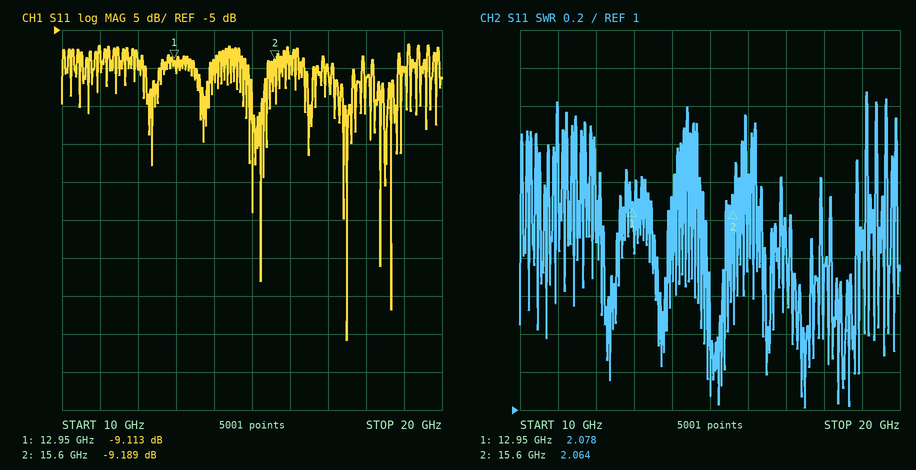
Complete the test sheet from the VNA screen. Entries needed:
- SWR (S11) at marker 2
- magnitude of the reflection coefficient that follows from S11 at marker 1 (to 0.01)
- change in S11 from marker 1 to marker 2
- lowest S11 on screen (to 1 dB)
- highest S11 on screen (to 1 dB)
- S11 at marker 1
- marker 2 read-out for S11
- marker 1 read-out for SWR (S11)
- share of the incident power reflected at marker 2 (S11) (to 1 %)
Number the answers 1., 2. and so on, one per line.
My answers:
1. 2.064
2. 0.35
3. -0.076 dB
4. -46 dB
5. -7 dB
6. -9.113 dB
7. -9.189 dB
8. 2.078
9. 12 %
